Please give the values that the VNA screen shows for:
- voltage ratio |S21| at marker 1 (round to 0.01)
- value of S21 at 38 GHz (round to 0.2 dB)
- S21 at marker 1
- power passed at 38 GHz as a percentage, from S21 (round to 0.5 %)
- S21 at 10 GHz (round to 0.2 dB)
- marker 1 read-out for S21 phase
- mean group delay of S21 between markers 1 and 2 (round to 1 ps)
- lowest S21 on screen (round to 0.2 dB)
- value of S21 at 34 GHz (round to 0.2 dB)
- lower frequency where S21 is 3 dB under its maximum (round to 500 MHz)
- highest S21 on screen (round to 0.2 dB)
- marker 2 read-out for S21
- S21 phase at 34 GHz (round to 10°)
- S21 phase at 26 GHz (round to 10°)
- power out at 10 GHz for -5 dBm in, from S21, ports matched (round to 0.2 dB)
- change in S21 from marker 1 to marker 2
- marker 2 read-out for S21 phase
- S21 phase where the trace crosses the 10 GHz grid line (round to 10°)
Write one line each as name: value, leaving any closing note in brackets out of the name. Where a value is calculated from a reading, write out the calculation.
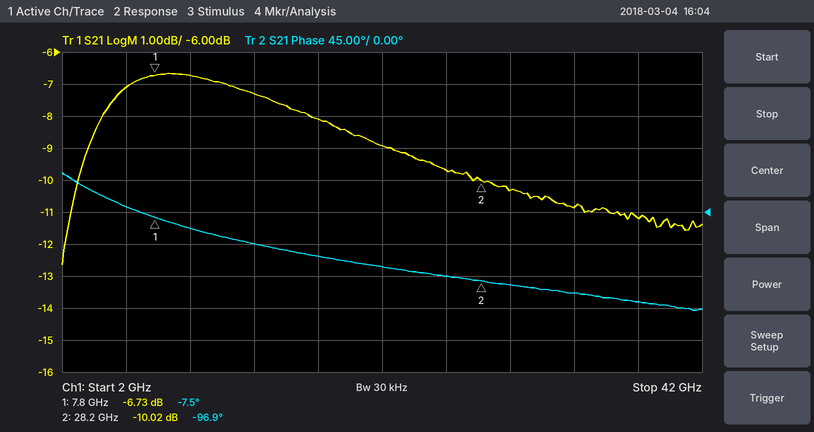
voltage ratio |S21| at marker 1: 10^(-6.73/20) ≈ 0.46
value of S21 at 38 GHz: -11.2 dB
S21 at marker 1: -6.73 dB
power passed at 38 GHz as a percentage, from S21: 10^(-11.2/10) ≈ 7.59 %, so 7.5 % to the nearest 0.5 %
S21 at 10 GHz: -6.8 dB
marker 1 read-out for S21 phase: -7.5°
mean group delay of S21 between markers 1 and 2: −(-96.9° − (-7.5°))/(360° × 20.4 GHz) ≈ 12 ps
lowest S21 on screen: -12.6 dB
value of S21 at 34 GHz: -10.8 dB
lower frequency where S21 is 3 dB under its maximum: 3.0 GHz
highest S21 on screen: -6.6 dB
marker 2 read-out for S21: -10.02 dB
S21 phase at 34 GHz: -110°
S21 phase at 26 GHz: -90°
power out at 10 GHz for -5 dBm in, from S21, ports matched: -5 dBm + (-6.8 dB) = -11.8 dBm
change in S21 from marker 1 to marker 2: -10.02 − (-6.73) = -3.29 dB
marker 2 read-out for S21 phase: -96.9°
S21 phase where the trace crosses the 10 GHz grid line: -20°
